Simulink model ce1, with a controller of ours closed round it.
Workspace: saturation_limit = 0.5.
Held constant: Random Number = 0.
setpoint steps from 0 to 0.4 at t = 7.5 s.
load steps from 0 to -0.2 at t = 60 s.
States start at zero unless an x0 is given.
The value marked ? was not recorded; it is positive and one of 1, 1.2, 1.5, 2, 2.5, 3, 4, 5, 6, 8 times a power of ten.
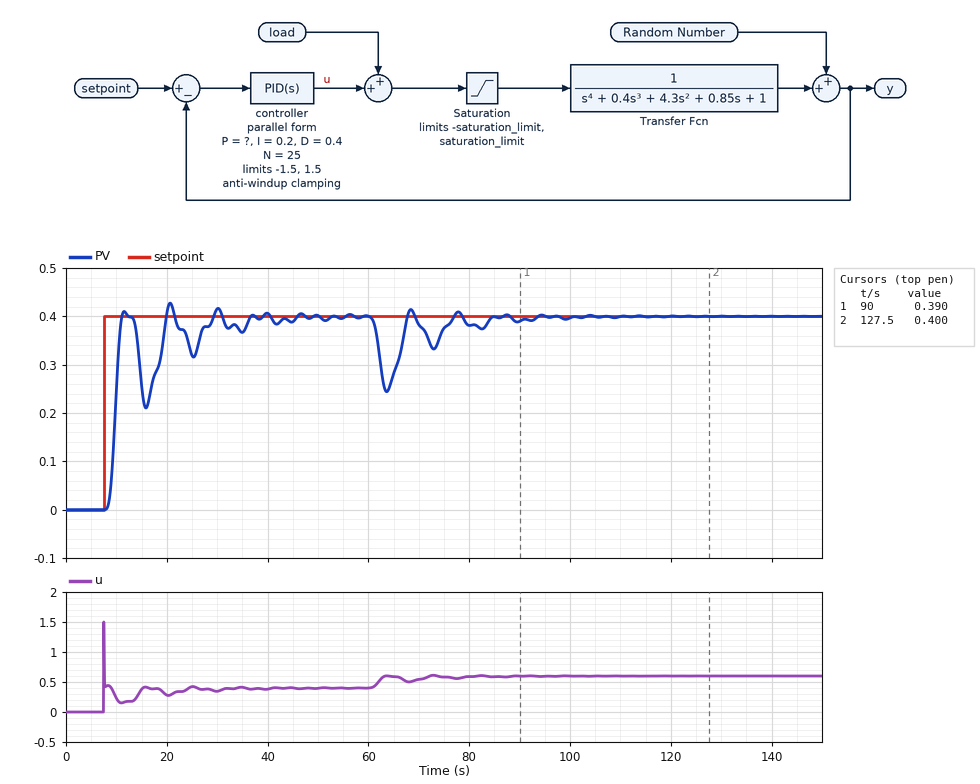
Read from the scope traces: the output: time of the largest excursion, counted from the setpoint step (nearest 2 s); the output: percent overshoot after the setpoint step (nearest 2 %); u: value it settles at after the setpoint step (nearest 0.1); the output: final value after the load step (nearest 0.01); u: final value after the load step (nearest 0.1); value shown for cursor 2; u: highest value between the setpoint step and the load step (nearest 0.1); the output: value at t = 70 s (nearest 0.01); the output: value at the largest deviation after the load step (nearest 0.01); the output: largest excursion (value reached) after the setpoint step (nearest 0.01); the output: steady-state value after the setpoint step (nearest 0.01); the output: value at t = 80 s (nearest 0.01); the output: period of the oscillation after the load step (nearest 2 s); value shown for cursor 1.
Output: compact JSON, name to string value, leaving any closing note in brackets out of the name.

{"the output: time of the largest excursion, counted from the setpoint step": "14 s", "the output: percent overshoot after the setpoint step": "6 %", "u: value it settles at after the setpoint step": "0.4", "the output: final value after the load step": "0.40", "u: final value after the load step": "0.6", "value shown for cursor 2": "0.400", "u: highest value between the setpoint step and the load step": "1.5", "the output: value at t = 70 s": "0.38", "the output: value at the largest deviation after the load step": "0.24", "the output: largest excursion (value reached) after the setpoint step": "0.43", "the output: steady-state value after the setpoint step": "0.40", "the output: value at t = 80 s": "0.38", "the output: period of the oscillation after the load step": "10 s", "value shown for cursor 1": "0.390"}
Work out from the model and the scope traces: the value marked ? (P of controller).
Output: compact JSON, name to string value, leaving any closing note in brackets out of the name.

{"the value marked ?": "1"}
